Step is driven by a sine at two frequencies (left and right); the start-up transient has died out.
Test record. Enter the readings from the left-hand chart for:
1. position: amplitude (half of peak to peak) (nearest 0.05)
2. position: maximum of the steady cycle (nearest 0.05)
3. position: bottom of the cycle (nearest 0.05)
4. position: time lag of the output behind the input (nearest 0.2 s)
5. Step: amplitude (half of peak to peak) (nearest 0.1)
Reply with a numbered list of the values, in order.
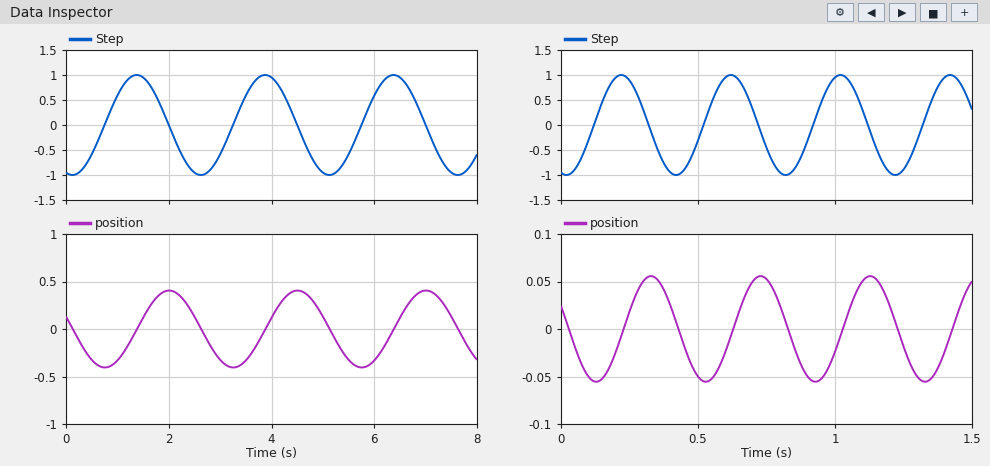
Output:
1. 0.40
2. 0.40
3. -0.40
4. 0.6 s
5. 1.0
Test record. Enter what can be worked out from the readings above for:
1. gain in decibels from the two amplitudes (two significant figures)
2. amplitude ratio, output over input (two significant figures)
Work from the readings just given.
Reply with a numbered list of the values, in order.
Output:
1. -8.0 dB
2. 0.40
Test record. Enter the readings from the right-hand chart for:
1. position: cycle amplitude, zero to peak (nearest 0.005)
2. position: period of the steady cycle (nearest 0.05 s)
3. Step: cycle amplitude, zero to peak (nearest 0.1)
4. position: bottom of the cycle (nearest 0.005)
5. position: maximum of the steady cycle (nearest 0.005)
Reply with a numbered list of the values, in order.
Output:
1. 0.055
2. 0.40 s
3. 1.0
4. -0.055
5. 0.055
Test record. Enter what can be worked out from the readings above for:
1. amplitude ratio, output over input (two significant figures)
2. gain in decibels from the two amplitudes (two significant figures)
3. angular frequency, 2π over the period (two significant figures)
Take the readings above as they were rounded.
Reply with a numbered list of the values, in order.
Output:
1. 0.055
2. -25 dB
3. 16 rad/s
